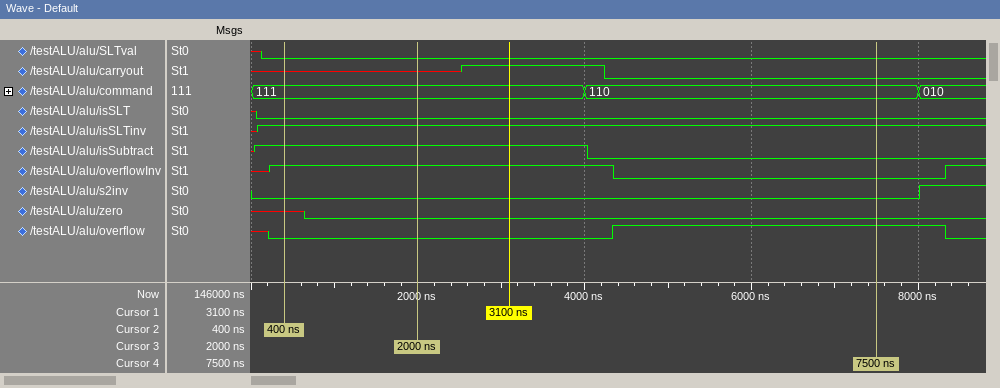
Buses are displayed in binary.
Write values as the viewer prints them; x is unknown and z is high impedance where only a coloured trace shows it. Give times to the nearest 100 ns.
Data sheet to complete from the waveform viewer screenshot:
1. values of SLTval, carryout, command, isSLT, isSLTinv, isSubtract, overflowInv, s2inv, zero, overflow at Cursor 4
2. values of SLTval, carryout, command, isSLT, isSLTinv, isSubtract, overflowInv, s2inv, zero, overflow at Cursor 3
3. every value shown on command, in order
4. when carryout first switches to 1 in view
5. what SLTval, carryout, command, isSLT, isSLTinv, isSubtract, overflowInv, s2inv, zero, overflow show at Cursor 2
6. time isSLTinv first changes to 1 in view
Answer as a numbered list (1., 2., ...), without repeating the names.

1. SLTval=0, carryout=0, command=110, isSLT=0, isSLTinv=1, isSubtract=0, overflowInv=0, s2inv=0, zero=0, overflow=1
2. SLTval=0, carryout=x, command=111, isSLT=0, isSLTinv=1, isSubtract=1, overflowInv=1, s2inv=0, zero=0, overflow=0
3. 111, 110, 010
4. 2500 ns
5. SLTval=0, carryout=x, command=111, isSLT=0, isSLTinv=1, isSubtract=1, overflowInv=1, s2inv=0, zero=x, overflow=0
6. 100 ns
